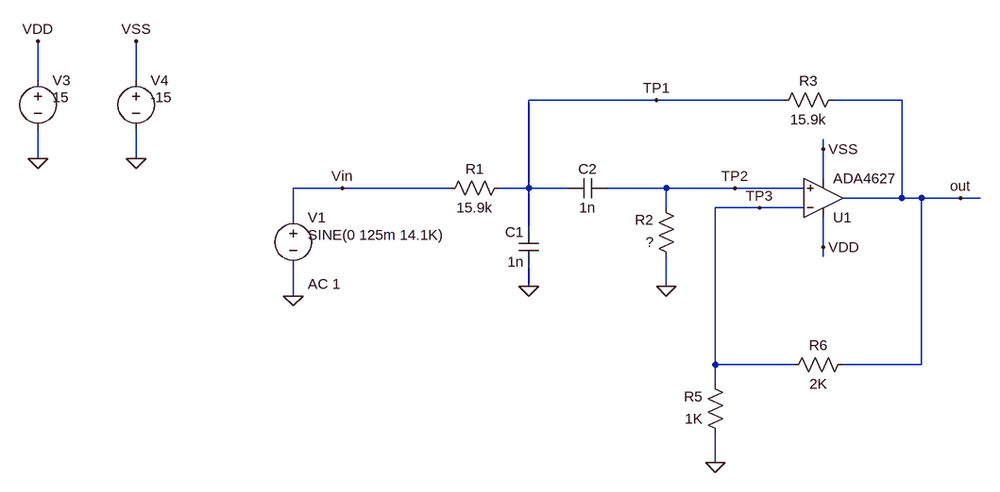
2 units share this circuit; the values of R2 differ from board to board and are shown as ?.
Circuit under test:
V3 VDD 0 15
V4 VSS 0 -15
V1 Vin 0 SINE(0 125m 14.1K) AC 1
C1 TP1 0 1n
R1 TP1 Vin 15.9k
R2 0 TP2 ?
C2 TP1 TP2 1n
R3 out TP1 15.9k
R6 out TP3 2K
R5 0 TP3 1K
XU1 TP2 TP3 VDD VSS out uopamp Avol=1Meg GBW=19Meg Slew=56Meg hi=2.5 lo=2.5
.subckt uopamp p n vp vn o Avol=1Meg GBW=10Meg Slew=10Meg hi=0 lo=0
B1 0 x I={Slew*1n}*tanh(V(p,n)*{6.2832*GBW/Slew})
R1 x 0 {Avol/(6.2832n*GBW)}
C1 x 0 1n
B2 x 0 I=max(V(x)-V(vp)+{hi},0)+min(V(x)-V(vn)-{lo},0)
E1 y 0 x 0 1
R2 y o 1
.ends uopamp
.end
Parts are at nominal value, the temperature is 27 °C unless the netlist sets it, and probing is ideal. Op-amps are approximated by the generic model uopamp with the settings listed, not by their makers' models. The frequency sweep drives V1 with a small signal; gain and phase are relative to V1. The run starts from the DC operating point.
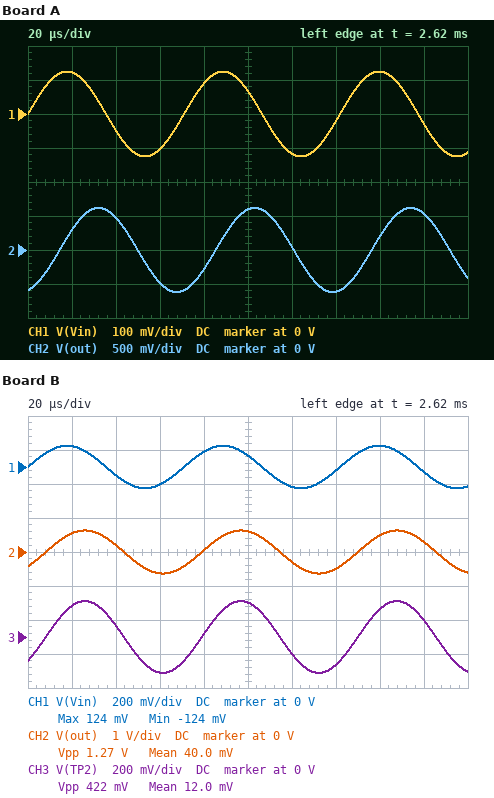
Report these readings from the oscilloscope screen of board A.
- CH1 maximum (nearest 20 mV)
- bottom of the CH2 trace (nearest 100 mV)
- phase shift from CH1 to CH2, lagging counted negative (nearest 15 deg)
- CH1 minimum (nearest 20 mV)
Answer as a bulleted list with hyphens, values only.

- 120 mV
- -600 mV
- -75 deg
- -120 mV
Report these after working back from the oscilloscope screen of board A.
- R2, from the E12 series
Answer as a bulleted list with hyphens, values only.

- 27 kΩ
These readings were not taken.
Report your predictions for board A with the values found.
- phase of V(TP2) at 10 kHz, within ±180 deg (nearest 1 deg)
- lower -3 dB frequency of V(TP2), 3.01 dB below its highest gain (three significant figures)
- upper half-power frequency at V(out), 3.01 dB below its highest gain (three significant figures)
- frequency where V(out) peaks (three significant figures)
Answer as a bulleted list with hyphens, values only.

- 45 deg
- 9.99 kHz
- 11.8 kHz
- 10.8 kHz
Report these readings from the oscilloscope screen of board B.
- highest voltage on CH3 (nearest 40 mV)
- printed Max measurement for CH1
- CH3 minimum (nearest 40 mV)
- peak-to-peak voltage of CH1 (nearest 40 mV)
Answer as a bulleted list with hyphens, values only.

- 200 mV
- 124 mV
- -200 mV
- 240 mV
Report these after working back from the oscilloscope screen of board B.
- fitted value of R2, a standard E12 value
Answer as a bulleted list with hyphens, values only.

- 22 kΩ
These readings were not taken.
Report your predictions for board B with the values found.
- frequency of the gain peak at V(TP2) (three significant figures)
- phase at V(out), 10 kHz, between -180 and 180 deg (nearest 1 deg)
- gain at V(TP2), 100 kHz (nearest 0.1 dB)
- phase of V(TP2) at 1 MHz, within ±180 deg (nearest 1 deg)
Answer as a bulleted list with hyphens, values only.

- 12.0 kHz
- 45 deg
- -19.9 dB
- -90 deg
